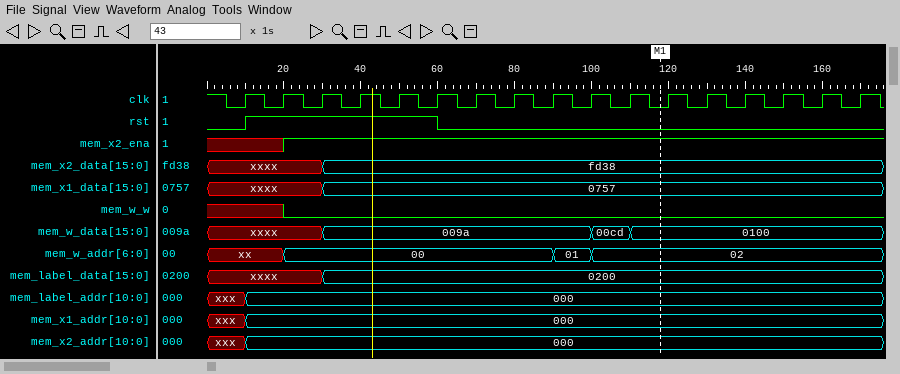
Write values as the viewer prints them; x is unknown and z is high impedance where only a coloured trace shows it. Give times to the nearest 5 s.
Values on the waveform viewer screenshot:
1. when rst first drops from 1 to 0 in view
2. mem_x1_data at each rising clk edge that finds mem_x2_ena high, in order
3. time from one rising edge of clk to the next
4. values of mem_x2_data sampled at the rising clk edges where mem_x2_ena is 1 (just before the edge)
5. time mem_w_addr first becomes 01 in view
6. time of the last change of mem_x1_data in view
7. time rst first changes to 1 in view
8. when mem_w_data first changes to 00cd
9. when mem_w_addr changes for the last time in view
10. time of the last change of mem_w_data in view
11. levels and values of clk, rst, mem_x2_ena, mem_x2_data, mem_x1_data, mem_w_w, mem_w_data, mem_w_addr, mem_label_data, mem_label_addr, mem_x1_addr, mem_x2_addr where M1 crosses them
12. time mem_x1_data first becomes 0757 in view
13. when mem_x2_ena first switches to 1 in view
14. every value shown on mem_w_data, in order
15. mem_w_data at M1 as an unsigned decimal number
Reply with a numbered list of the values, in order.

1. 60 s
2. xxxx, 0757, 0757, 0757, 0757, 0757, 0757, 0757, 0757, 0757, 0757, 0757, 0757, 0757, 0757
3. 10 s
4. xxxx, fd38, fd38, fd38, fd38, fd38, fd38, fd38, fd38, fd38, fd38, fd38, fd38, fd38, fd38
5. 90 s
6. 30 s
7. 10 s
8. 100 s
9. 100 s
10. 110 s
11. clk=0, rst=0, mem_x2_ena=1, mem_x2_data=fd38, mem_x1_data=0757, mem_w_w=0, mem_w_data=0100, mem_w_addr=02, mem_label_data=0200, mem_label_addr=000, mem_x1_addr=000, mem_x2_addr=000
12. 30 s
13. 20 s
14. xxxx, 009a, 00cd, 0100
15. 256
